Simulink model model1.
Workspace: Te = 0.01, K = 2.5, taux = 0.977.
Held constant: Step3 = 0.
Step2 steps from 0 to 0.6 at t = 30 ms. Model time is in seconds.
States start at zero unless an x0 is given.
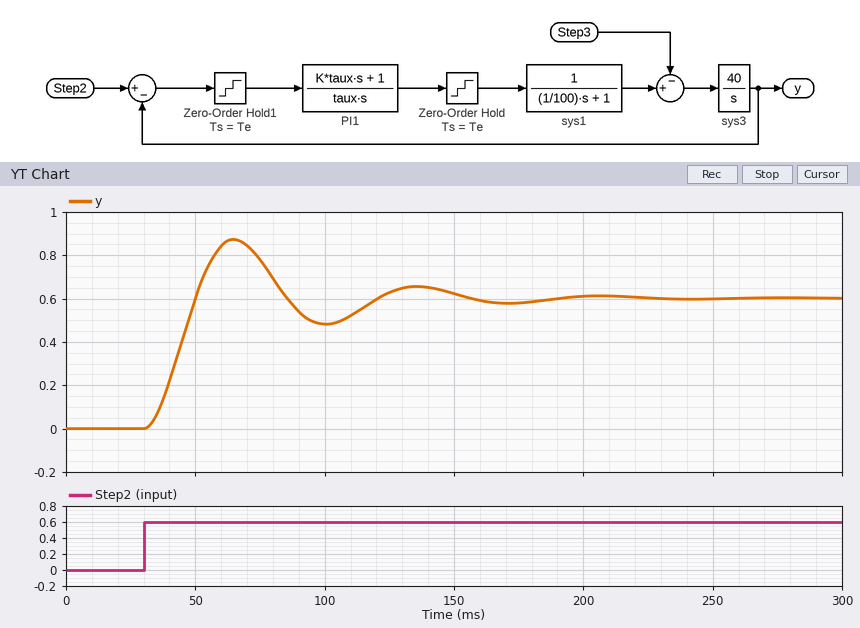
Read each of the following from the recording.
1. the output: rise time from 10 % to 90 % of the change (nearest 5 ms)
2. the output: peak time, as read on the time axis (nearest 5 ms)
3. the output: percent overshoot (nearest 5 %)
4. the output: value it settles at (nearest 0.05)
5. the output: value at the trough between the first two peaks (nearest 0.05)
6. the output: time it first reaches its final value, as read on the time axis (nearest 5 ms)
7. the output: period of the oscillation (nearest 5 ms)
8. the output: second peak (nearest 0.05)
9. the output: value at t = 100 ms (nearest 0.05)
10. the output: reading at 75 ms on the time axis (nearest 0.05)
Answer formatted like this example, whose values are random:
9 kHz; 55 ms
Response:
15 ms; 65 ms; 45 %; 0.60; 0.50; 50 ms; 70 ms; 0.65; 0.50; 0.80
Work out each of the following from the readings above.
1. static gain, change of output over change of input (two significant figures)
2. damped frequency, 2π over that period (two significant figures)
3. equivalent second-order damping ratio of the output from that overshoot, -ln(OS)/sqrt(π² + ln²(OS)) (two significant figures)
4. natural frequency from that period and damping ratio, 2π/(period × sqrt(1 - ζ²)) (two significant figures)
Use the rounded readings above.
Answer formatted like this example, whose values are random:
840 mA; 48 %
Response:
1.0; 0.090 rad/ms; 0.25; 0.093 rad/ms
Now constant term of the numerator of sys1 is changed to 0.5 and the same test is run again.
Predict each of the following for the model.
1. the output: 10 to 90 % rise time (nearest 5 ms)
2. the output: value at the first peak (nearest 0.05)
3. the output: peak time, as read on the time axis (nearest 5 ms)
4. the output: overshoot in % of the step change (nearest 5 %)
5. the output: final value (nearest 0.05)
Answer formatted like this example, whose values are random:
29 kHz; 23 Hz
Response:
25 ms; 0.70; 85 ms; 15 %; 0.60
